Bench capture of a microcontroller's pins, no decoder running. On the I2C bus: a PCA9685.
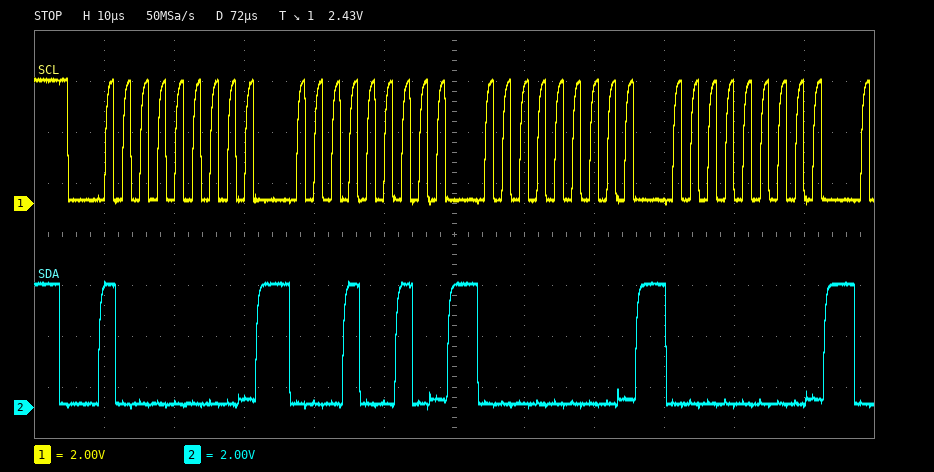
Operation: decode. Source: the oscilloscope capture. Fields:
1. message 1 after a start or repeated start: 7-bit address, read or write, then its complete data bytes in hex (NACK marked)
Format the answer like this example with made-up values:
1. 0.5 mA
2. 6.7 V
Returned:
1. 0x40 write: 12 00 00
